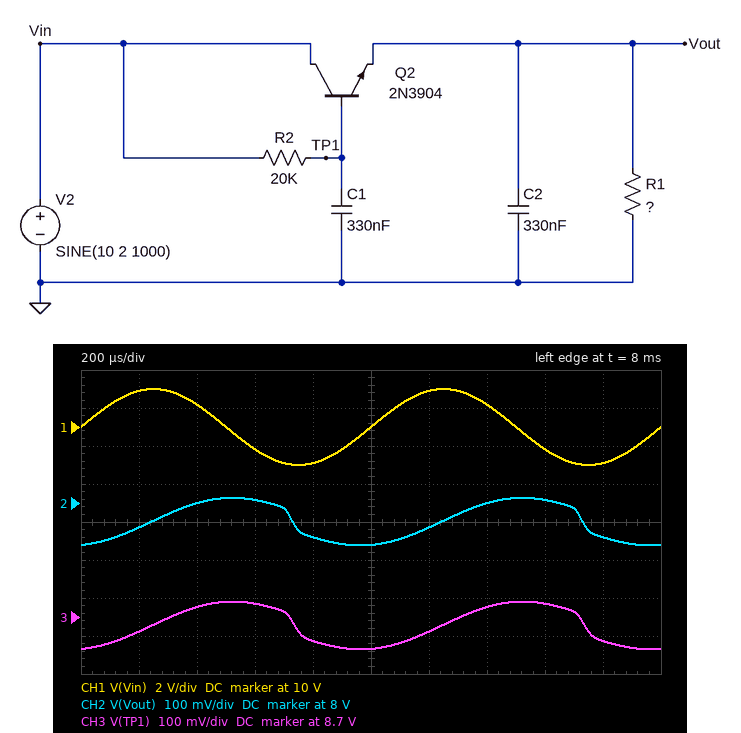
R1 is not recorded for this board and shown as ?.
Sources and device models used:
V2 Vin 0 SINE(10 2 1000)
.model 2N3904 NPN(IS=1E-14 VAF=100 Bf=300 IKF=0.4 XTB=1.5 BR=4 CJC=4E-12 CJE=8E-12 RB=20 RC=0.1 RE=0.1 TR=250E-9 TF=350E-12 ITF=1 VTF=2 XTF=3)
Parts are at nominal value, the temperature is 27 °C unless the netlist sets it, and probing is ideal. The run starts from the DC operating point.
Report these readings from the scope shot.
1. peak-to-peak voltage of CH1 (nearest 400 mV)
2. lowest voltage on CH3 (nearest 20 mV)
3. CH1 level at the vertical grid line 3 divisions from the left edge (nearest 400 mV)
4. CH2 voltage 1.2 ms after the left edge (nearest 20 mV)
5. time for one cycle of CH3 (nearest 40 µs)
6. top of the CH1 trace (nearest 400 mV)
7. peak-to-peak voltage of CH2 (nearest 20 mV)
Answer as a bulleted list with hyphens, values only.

- 4.0 V
- 8.62 V
- 8.8 V
- 7.94 V
- 1.00 ms
- 12.0 V
- 120 mV
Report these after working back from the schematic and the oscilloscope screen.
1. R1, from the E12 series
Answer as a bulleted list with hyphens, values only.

- 560 Ω
